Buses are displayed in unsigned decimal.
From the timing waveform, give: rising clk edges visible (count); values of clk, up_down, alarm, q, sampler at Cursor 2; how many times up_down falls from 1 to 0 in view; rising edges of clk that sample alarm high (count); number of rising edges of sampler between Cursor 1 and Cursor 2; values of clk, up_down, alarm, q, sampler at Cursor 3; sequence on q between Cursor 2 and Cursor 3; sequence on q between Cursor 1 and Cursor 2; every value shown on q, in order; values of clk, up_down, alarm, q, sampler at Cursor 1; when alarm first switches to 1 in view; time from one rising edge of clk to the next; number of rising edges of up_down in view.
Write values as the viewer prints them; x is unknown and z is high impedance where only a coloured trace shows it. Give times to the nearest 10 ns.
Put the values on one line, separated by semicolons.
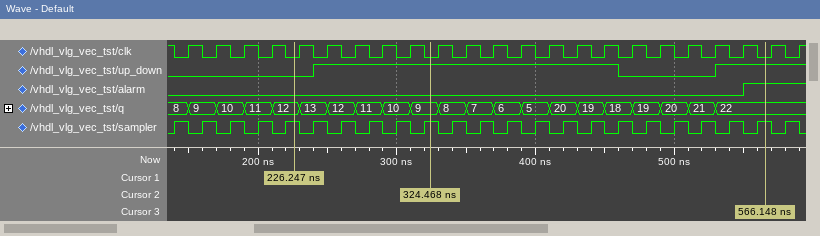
23; clk=0, up_down=1, alarm=0, q=9, sampler=1; 1; 2; 5; clk=0, up_down=1, alarm=1, q=22, sampler=1; 9, 8, 7, 6, 5, 20, 19, 18, 19, 20, 21, 22; 12, 13, 12, 11, 10, 9; 8, 9, 10, 11, 12, 13, 12, 11, 10, 9, 8, 7, 6, 5, 20, 19, 18, 19, 20, 21, 22; clk=0, up_down=0, alarm=0, q=12, sampler=1; 550 ns; 20 ns; 2
